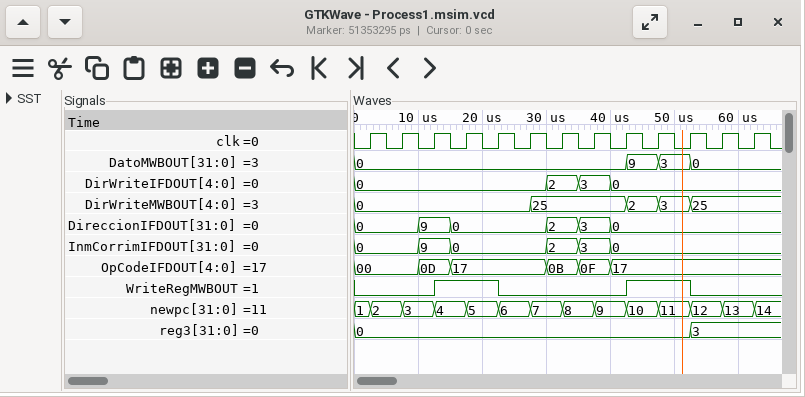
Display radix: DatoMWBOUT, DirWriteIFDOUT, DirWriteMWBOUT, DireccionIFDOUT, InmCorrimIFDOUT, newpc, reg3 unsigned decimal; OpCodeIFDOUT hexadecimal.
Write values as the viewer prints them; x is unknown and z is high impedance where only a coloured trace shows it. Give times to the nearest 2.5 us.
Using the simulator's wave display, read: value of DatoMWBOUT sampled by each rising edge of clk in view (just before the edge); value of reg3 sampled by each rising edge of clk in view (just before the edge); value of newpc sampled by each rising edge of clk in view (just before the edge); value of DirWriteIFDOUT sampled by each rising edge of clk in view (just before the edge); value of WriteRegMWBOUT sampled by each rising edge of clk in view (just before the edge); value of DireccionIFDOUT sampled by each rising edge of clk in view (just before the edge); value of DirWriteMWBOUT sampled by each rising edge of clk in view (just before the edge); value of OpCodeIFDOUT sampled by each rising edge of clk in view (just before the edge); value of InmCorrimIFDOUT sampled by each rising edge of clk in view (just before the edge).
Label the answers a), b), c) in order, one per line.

a) 0, 0, 0, 0, 0, 0, 0, 0, 0, 9, 3, 0, 0
b) 0, 0, 0, 0, 0, 0, 0, 0, 0, 0, 0, 3, 3
c) 1, 2, 3, 4, 5, 6, 7, 8, 9, 10, 11, 12, 13
d) 0, 0, 0, 0, 0, 0, 2, 3, 0, 0, 0, 0, 0
e) 0 0 0 1 1 0 0 0 0 1 1 0 0
f) 0, 0, 9, 0, 0, 0, 2, 3, 0, 0, 0, 0, 0
g) 0, 0, 0, 0, 0, 0, 25, 25, 25, 2, 3, 25, 25
h) 00, 00, 0D, 17, 17, 17, 0B, 0F, 17, 17, 17, 17, 17
i) 0, 0, 9, 0, 0, 0, 2, 3, 0, 0, 0, 0, 0
